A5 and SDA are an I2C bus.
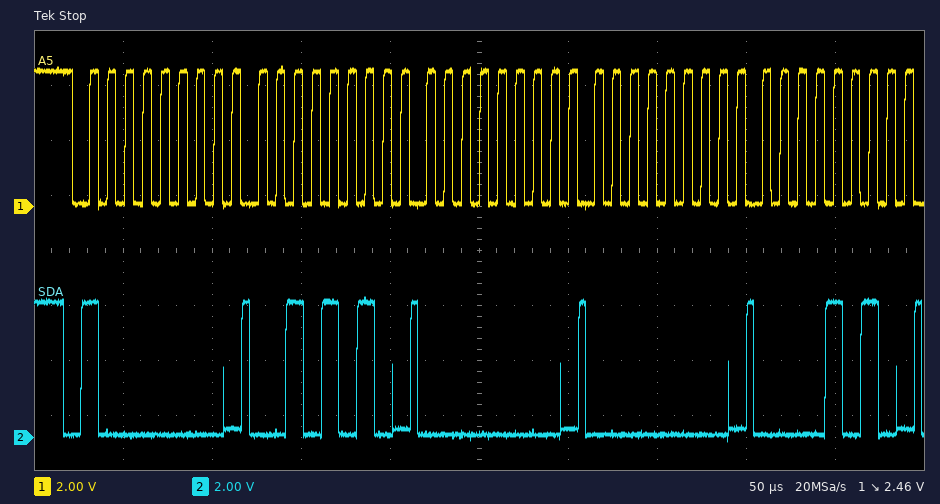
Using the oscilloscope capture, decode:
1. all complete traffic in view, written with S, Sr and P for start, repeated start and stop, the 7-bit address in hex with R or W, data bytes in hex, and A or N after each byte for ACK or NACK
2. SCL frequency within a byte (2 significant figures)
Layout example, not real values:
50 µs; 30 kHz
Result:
S 40W A 2A A 00 A 00 A 0A A; 100 kHz
